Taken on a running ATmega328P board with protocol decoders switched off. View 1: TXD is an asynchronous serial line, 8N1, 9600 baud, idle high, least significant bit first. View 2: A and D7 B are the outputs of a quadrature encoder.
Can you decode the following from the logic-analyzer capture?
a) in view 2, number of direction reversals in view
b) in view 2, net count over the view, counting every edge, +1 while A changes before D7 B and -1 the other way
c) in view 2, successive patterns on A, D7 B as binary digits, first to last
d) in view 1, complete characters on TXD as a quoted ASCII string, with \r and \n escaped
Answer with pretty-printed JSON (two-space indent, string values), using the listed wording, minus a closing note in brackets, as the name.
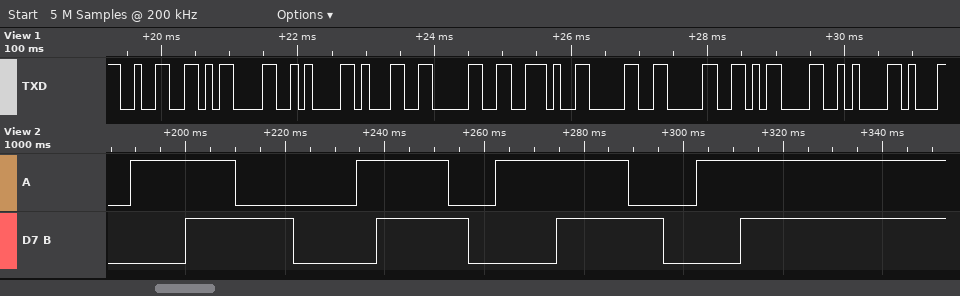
{
  "in view 2, number of direction reversals in view": "0",
  "in view 2, net count over the view, counting every edge, +1 while A changes before D7 B and -1 the other way": "+14",
  "in view 2, successive patterns on A, D7 B as binary digits, first to last": "00 10 11 01 00 10 11 01 00 10 11 01 00 10 11",
  "in view 1, complete characters on TXD as a quoted ASCII string, with \\r and \\n escaped": "\"2\\r\\n10.00\\r\\n\""
}
